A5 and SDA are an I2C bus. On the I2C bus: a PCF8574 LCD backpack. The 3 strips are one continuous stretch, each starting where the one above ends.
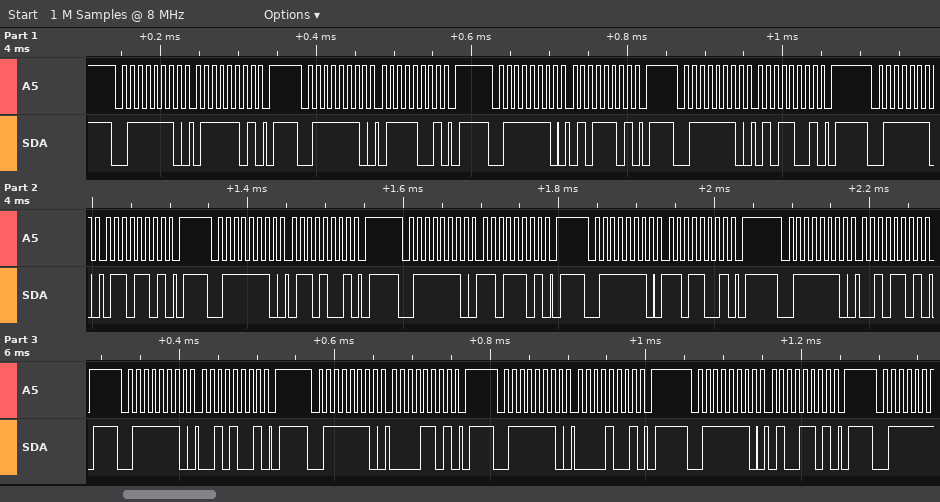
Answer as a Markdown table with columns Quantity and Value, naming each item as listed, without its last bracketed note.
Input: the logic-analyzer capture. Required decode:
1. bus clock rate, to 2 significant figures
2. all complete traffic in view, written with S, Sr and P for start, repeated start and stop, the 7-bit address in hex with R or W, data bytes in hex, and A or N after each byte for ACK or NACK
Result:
| Quantity | Value |
|---|---|
| bus clock rate, to 2 significant figures | 100 kHz |
| all complete traffic in view, written with S, Sr and P for start, repeated start and stop, the 7-bit address in hex with R or W, data bytes in hex, and A or N after each byte for ACK or NACK | S 3FW A 7D A P S 3FW A 79 A P S 3FW A 5D A P S 3FW A 59 A P S 3FW A 6D A P S 3FW A 69 A P S 3FW A DD A P S 3FW A D9 A P S 3FW A 2D A P S 3FW A 29 A P S 3FW A 0D A P S 3FW A 09 A P S 3FW A 4D A P |
